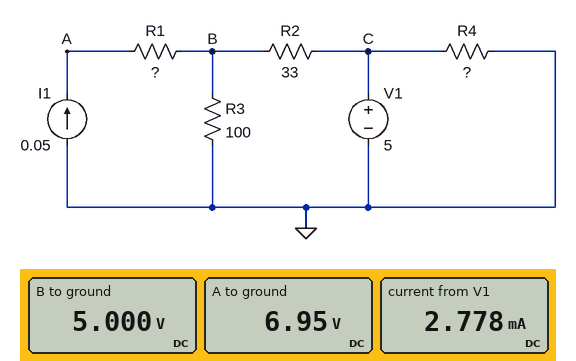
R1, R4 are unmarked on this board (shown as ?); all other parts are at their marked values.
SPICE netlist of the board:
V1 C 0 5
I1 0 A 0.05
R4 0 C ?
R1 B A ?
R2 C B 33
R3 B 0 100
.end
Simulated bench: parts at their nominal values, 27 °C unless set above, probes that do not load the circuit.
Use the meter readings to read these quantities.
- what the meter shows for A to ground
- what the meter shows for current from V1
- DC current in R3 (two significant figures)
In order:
6.95 V
2.778 mA
50 mA
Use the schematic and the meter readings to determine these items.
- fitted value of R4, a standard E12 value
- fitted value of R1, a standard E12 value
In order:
1.8 kΩ
39 Ω
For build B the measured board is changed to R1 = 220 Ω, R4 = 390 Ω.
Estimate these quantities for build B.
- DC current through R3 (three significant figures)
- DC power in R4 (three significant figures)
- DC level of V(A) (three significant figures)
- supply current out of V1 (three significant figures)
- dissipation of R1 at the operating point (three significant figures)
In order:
50.0 mA
64.1 mW
16.0 V
12.8 mA
550 mW
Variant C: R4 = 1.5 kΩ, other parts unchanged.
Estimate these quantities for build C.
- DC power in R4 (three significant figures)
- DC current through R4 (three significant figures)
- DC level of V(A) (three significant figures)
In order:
16.7 mW
3.33 mA
6.95 V
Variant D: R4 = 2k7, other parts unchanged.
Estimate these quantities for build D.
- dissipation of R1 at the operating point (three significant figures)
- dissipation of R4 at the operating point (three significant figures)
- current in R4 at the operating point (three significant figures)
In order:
97.5 mW
9.26 mW
1.85 mA
